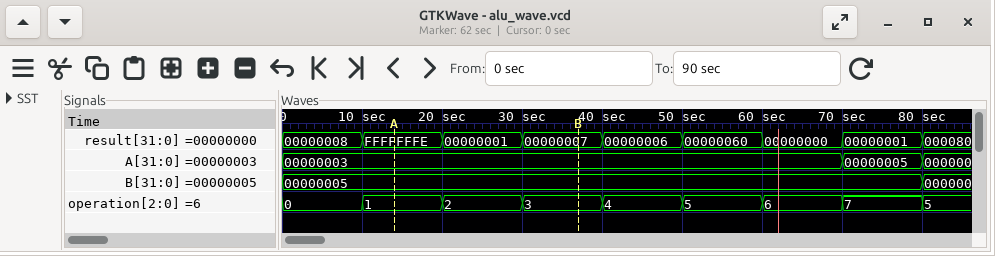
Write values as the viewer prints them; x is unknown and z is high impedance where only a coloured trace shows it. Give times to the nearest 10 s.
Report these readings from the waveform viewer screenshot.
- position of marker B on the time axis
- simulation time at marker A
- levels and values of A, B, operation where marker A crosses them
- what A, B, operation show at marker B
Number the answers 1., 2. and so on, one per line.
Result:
1. 40 s
2. 10 s
3. A=00000003, B=00000005, operation=1
4. A=00000003, B=00000005, operation=3
